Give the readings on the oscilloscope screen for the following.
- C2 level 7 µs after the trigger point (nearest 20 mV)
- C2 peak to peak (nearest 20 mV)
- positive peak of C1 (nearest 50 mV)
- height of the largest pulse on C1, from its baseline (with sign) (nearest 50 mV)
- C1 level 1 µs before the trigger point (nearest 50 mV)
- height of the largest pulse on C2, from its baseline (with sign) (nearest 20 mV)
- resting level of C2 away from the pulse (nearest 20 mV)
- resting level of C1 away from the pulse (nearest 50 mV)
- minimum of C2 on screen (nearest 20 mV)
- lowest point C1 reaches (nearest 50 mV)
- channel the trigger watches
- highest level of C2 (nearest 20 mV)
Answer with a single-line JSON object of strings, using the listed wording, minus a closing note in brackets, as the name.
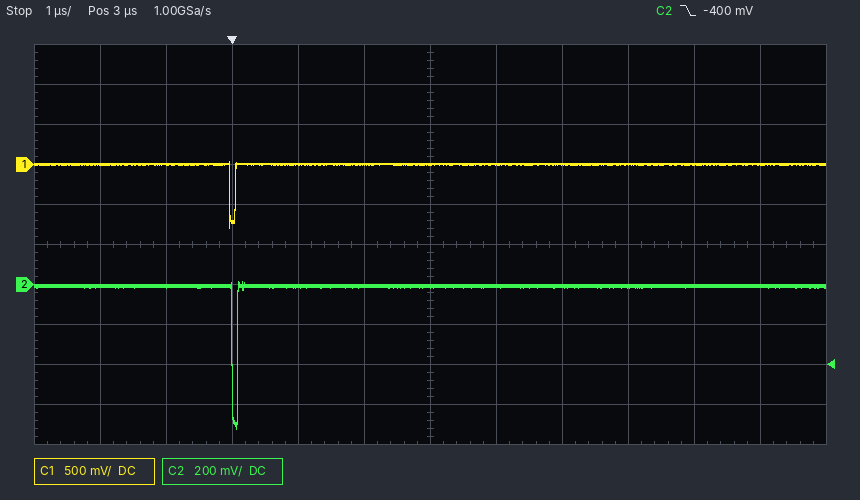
{"C2 level 7 µs after the trigger point": "0 mV", "C2 peak to peak": "740 mV", "positive peak of C1": "50 mV", "height of the largest pulse on C1, from its baseline (with sign)": "-800 mV", "C1 level 1 µs before the trigger point": "0 mV", "height of the largest pulse on C2, from its baseline (with sign)": "-720 mV", "resting level of C2 away from the pulse": "0 mV", "resting level of C1 away from the pulse": "0 mV", "minimum of C2 on screen": "-720 mV", "lowest point C1 reaches": "-800 mV", "channel the trigger watches": "C2", "highest level of C2": "20 mV"}
